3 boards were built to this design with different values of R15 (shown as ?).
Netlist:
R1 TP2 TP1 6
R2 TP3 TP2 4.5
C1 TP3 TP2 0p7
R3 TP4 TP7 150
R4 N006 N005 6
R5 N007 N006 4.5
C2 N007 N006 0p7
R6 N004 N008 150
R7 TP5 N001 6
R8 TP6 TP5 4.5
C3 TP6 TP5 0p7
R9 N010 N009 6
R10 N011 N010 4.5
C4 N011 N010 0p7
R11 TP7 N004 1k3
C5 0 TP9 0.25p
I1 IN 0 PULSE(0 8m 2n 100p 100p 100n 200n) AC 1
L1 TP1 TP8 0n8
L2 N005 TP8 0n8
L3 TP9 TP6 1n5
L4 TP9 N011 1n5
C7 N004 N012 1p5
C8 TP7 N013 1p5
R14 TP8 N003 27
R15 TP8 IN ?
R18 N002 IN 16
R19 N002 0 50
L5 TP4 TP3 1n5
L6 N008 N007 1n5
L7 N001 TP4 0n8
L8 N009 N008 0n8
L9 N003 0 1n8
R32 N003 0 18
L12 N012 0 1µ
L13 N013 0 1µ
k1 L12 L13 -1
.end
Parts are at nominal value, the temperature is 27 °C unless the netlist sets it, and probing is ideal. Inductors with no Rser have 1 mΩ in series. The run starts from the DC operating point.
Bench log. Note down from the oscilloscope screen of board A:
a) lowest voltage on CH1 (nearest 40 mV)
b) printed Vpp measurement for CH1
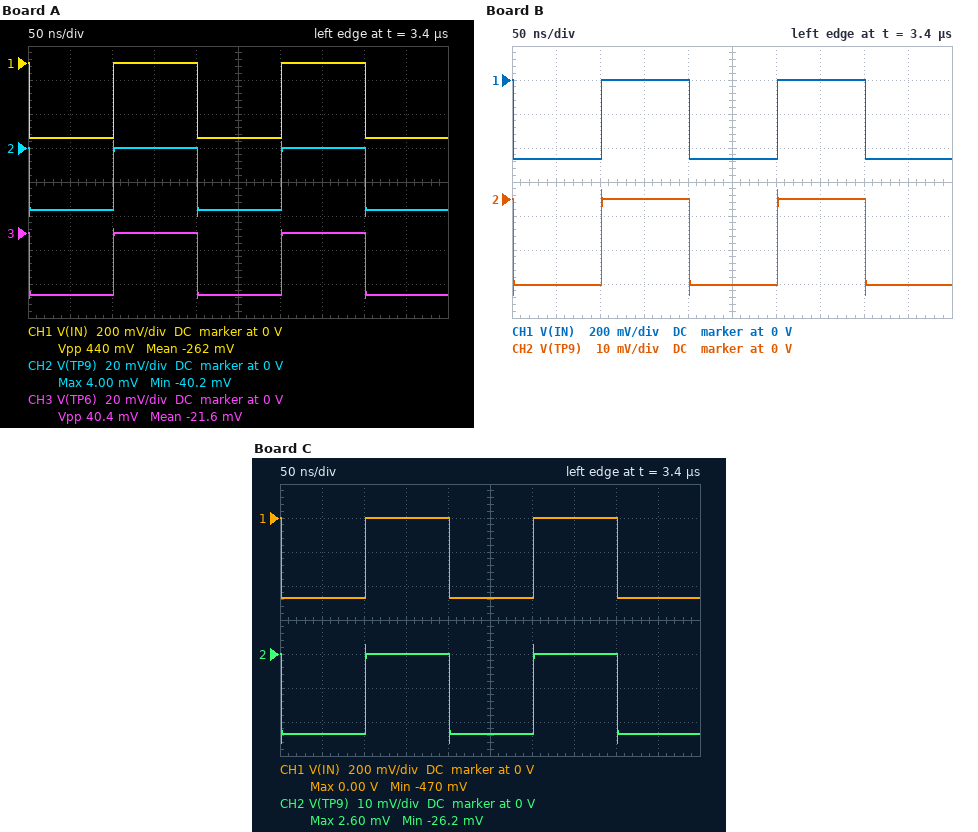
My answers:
-440 mV
440 mV
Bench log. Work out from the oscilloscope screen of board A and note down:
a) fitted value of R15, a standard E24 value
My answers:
300 Ω
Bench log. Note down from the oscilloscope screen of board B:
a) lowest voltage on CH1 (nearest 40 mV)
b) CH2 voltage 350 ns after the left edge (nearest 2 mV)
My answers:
-480 mV
0 V
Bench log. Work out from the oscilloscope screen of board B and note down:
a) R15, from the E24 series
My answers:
470 Ω
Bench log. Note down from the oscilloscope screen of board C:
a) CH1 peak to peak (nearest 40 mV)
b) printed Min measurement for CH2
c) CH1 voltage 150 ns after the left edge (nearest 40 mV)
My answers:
480 mV
-26.2 mV
0 V
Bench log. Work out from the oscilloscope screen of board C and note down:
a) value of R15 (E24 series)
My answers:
510 Ω
